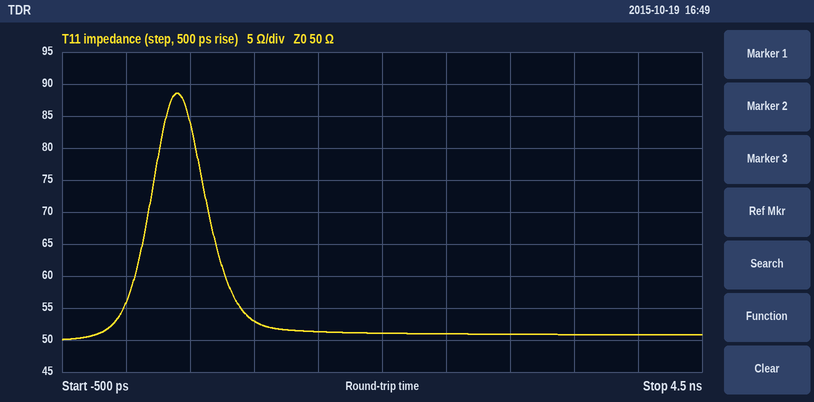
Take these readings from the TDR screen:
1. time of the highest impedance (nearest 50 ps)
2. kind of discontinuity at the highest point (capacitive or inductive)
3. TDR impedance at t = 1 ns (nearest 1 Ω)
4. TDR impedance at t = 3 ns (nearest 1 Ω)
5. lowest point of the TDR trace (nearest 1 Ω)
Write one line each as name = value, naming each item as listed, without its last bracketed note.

time of the highest impedance = 400 ps
kind of discontinuity at the highest point = inductive
TDR impedance at t = 1 ns = 53 Ω
TDR impedance at t = 3 ns = 51 Ω
lowest point of the TDR trace = 50 Ω
